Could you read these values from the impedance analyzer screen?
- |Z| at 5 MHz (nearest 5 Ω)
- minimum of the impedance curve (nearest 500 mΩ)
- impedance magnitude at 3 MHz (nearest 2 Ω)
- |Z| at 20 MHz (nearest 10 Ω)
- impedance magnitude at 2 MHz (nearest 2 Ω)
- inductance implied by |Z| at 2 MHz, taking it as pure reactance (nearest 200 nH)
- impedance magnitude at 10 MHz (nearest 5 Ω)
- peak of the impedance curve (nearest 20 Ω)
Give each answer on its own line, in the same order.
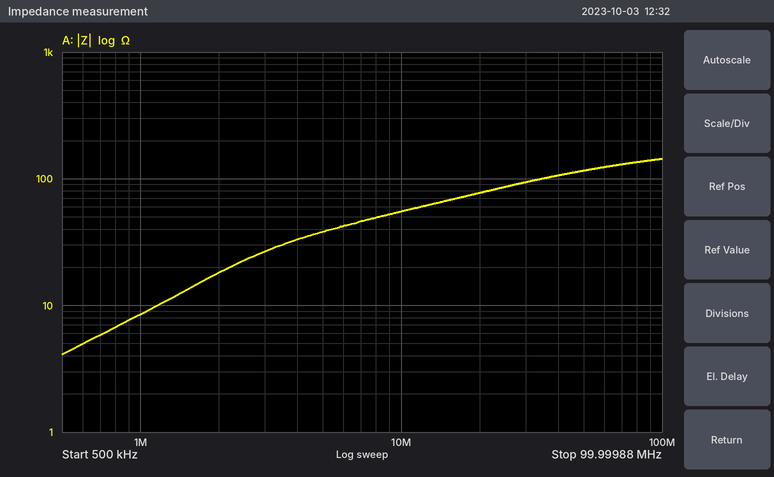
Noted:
40 Ω
4.0 Ω
26 Ω
80 Ω
18 Ω
1.4 µH
55 Ω
140 Ω
